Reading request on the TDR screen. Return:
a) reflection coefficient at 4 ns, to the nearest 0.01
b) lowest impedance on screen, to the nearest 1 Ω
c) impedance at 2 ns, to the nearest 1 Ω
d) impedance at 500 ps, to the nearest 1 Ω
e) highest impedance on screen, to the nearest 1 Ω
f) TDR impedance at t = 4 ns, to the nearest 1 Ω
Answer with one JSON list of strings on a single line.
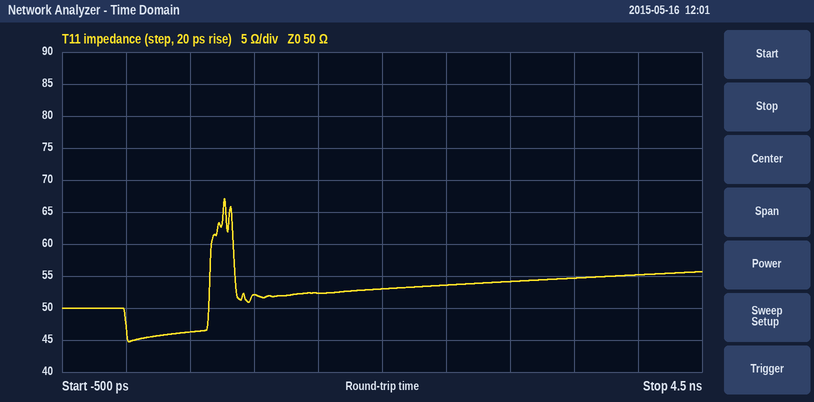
["+0.05", "45 Ω", "53 Ω", "46 Ω", "67 Ω", "55 Ω"]
